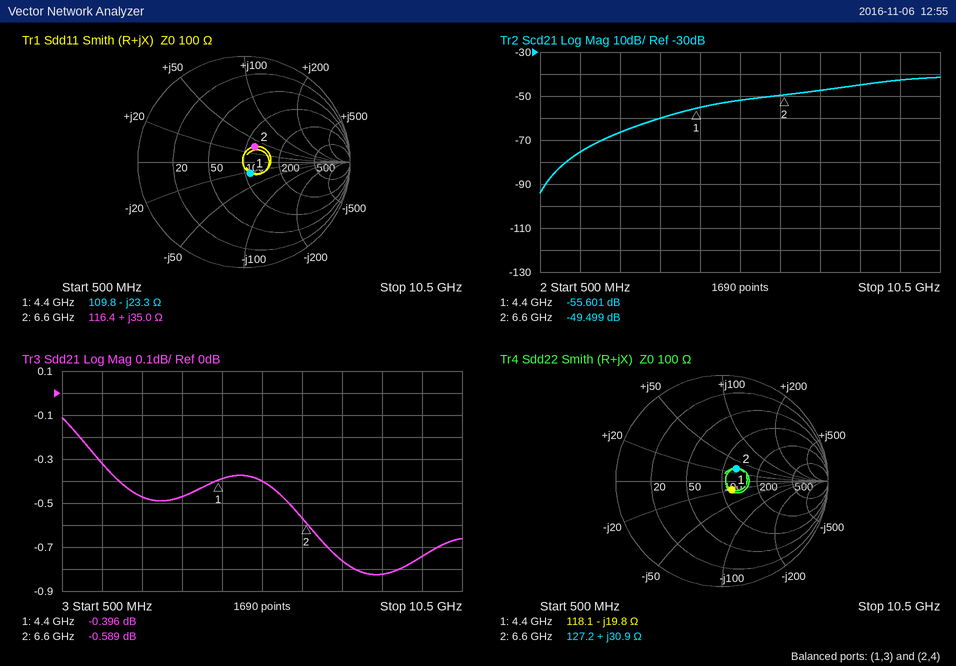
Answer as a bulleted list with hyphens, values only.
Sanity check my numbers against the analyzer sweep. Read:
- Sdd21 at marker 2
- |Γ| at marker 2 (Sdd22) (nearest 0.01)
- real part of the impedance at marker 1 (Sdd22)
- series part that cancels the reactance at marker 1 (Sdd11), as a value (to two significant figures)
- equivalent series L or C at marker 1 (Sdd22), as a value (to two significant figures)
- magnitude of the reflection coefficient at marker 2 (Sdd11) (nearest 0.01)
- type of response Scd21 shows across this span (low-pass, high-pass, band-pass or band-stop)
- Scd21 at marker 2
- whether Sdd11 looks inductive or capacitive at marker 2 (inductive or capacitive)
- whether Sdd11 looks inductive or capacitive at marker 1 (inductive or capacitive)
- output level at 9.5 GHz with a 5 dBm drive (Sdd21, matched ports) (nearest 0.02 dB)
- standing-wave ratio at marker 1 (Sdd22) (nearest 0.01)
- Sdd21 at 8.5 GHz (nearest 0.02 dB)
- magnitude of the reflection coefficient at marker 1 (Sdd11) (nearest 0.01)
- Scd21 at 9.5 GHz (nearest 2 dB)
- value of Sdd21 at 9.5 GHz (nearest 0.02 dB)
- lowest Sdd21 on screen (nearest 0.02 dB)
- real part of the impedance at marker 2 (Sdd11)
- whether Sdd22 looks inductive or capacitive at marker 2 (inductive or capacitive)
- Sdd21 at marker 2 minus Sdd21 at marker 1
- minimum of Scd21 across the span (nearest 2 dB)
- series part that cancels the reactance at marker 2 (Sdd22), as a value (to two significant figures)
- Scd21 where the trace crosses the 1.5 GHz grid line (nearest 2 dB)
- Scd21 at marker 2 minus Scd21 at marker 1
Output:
- -0.589 dB
- 0.18
- 118.1 Ω
- 840 pH
- 1.8 pF
- 0.18
- high-pass
- -49.499 dB
- inductive
- capacitive
- 4.26 dBm
- 1.28
- -0.82 dB
- 0.12
- -42 dB
- -0.74 dB
- -0.82 dB
- 116.4 Ω
- inductive
- -0.193 dB
- -94 dB
- 780 fF
- -76 dB
- 6.102 dB
